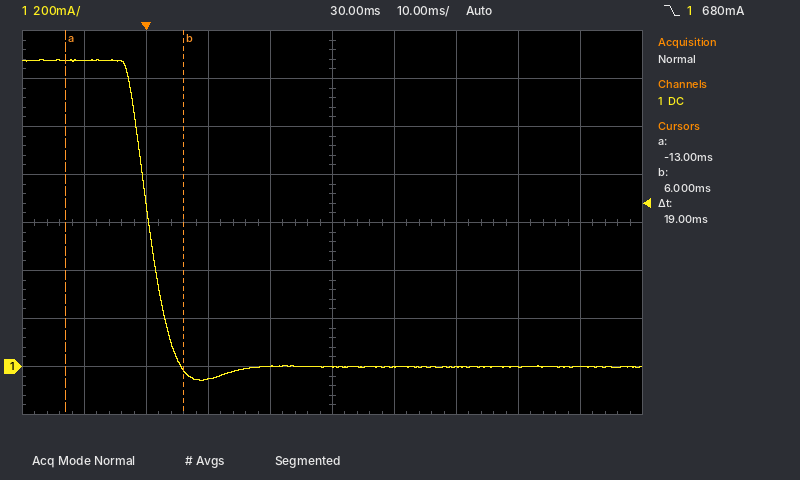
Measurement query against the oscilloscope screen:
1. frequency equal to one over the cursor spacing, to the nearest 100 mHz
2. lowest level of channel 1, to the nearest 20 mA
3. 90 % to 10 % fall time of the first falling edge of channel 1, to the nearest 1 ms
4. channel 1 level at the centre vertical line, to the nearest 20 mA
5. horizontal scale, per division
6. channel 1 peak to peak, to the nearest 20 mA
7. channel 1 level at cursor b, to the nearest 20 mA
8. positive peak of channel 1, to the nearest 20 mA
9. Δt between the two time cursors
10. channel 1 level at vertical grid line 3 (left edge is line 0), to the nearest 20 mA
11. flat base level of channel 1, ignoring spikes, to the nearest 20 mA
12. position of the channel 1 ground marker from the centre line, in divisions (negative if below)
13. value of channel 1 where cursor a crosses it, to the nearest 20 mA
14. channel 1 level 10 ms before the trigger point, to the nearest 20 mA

52.6 Hz
-60 mA
6 ms
0 mA
10 ms
1.34 A
-20 mA
1.28 A
19 ms
-60 mA
0 mA
-3.0 div
1.28 A
1.28 A
